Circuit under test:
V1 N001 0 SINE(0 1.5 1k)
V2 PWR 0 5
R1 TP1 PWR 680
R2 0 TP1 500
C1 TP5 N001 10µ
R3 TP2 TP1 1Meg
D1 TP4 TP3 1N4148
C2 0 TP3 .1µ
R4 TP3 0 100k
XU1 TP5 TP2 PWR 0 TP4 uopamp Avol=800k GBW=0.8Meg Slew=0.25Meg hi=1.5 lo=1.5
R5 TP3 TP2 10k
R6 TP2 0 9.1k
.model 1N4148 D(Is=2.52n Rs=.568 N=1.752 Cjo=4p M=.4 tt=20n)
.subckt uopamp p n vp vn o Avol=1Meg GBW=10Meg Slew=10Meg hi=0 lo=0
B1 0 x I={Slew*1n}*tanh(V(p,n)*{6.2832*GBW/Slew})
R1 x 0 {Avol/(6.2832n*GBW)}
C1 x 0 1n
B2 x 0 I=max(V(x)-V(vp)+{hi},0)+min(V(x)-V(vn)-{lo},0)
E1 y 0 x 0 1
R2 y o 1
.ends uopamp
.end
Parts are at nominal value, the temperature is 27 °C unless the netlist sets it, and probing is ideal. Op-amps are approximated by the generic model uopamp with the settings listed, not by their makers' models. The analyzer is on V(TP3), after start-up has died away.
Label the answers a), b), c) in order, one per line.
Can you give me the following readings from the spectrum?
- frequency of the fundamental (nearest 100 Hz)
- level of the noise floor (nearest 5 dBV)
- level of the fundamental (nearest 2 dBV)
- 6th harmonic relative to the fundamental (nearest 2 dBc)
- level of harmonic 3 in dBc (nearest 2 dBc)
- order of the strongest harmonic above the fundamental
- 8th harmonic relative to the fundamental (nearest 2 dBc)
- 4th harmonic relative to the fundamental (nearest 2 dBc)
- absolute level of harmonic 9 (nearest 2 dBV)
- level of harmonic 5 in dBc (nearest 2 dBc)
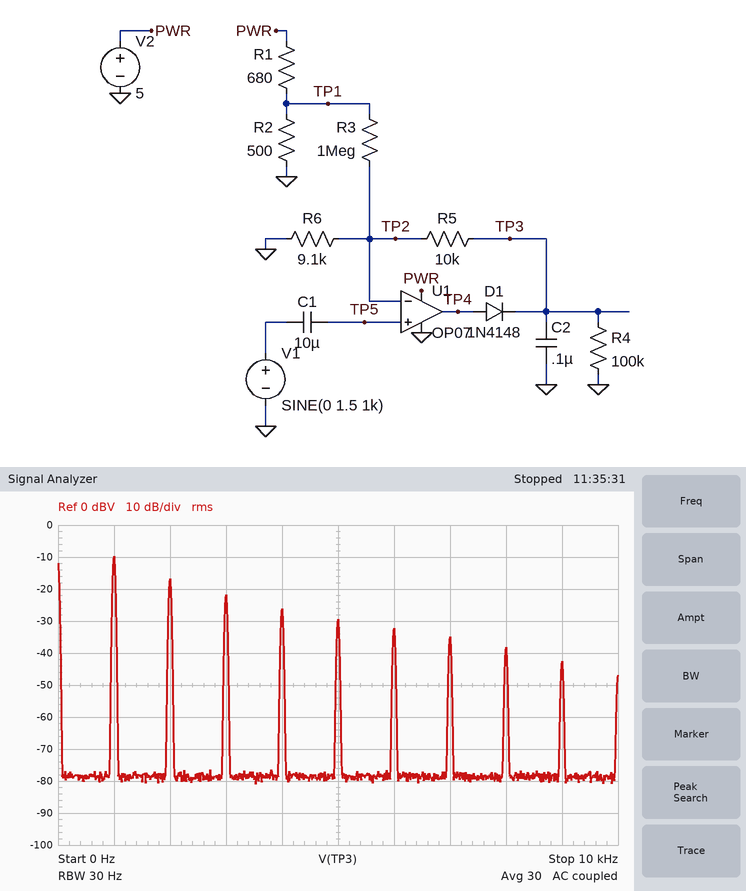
a) 1.0 kHz
b) -80 dBV
c) -10 dBV
d) -22 dBc
e) -12 dBc
f) 2
g) -28 dBc
h) -16 dBc
i) -42 dBV
j) -20 dBc
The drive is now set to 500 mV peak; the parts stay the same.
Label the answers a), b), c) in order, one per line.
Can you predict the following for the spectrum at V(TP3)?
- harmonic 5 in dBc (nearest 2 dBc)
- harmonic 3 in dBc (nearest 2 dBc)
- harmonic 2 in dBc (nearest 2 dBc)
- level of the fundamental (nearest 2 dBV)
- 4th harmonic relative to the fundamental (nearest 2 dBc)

a) -14 dBc
b) -6 dBc
c) -2 dBc
d) -90 dBV
e) -10 dBc
